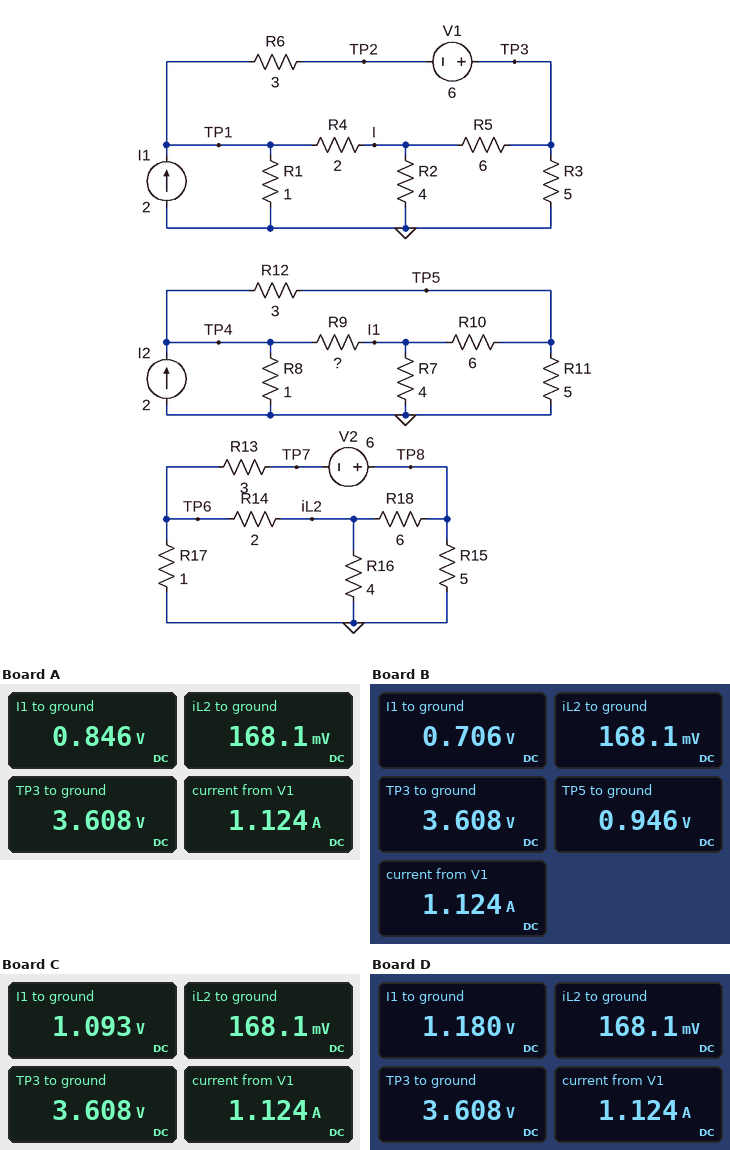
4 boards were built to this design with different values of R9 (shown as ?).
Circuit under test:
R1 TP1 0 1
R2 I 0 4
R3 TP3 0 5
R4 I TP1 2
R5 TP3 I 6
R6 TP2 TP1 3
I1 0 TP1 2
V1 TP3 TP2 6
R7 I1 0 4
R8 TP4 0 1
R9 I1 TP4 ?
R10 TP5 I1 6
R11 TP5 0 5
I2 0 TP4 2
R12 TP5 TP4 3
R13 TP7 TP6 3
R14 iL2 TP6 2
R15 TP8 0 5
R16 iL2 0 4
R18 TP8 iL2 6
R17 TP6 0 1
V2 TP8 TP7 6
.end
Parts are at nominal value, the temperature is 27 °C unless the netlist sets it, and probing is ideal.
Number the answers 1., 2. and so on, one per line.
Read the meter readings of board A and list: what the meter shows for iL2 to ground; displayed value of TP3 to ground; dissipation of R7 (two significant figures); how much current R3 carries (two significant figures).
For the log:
1. 168.1 mV
2. 3.608 V
3. 180 mW
4. 720 mA
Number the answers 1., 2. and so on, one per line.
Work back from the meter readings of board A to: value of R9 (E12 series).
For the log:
1. 3.9 Ω
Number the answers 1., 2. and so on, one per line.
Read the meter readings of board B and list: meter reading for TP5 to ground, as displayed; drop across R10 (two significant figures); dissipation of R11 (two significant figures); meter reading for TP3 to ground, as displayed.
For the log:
1. 0.946 V
2. 240 mV
3. 180 mW
4. 3.608 V
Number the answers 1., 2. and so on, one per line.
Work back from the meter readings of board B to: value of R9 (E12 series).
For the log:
1. 6.8 Ω
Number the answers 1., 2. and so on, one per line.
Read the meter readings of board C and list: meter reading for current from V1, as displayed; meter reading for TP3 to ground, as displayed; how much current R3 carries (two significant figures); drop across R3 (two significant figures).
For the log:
1. 1.124 A
2. 3.608 V
3. 720 mA
4. 3.6 V
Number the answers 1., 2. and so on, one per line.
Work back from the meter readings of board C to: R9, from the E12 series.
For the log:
1. 1.5 Ω
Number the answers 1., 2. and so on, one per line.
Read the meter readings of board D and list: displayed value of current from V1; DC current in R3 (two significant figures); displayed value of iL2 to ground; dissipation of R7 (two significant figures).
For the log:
1. 1.124 A
2. 720 mA
3. 168.1 mV
4. 350 mW
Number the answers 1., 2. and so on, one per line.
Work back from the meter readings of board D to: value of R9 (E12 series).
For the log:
1. 1 Ω
